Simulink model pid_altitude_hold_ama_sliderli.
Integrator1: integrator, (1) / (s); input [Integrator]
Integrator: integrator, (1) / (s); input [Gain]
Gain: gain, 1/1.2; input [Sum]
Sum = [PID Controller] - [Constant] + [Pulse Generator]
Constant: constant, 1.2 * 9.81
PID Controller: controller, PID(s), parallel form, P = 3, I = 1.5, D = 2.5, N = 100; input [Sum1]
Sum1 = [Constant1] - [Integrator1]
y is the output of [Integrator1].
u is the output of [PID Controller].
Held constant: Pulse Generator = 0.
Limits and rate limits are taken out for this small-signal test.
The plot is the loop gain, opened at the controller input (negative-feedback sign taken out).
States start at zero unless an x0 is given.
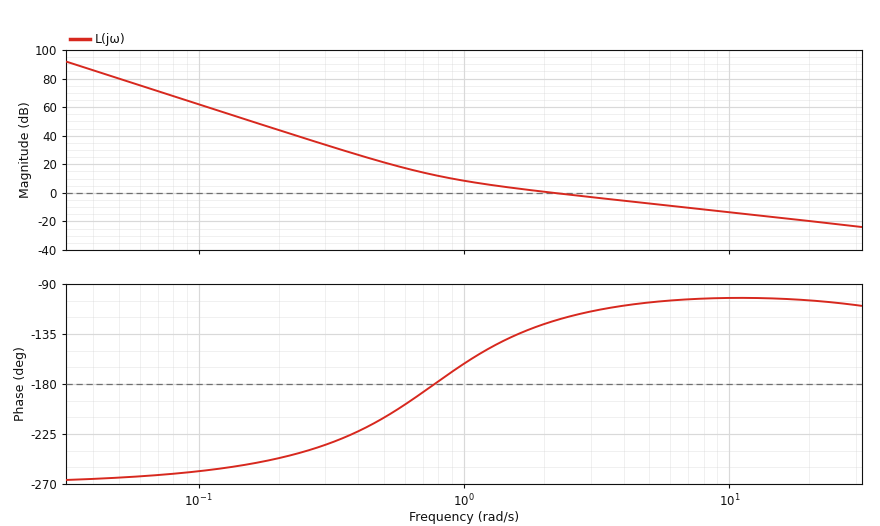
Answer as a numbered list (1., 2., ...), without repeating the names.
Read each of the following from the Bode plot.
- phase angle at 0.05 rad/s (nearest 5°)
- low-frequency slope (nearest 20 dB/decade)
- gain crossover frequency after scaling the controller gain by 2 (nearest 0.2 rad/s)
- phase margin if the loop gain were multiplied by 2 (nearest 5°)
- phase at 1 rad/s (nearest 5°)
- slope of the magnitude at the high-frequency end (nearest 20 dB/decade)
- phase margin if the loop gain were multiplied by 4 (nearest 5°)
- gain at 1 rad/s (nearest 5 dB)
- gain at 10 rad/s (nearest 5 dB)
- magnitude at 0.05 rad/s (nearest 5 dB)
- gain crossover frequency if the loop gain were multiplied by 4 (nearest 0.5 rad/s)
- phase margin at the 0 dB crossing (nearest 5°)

1. -265°
2. -60 dB/decade
3. 4.2 rad/s
4. 70°
5. -160°
6. -20 dB/decade
7. 75°
8. 10 dB
9. -15 dB
10. 80 dB
11. 8.5 rad/s
12. 55°
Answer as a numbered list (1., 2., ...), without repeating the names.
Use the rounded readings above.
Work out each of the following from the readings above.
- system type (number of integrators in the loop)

1. 3
